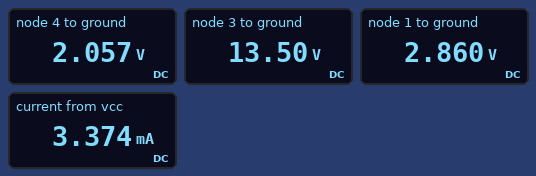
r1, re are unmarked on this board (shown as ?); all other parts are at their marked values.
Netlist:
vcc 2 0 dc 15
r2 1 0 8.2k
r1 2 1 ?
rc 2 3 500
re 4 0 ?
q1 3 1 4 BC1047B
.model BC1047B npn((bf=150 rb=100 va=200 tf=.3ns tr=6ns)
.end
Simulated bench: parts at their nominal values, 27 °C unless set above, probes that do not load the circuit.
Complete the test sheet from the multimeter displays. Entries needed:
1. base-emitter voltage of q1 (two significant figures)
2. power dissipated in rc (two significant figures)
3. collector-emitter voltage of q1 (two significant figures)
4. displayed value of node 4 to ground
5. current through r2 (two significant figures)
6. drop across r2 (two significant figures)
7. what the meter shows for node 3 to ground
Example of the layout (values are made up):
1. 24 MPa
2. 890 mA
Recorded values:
1. 800 mV
2. 4.5 mW
3. 11 V
4. 2.057 V
5. 350 µA
6. 2.9 V
7. 13.50 V
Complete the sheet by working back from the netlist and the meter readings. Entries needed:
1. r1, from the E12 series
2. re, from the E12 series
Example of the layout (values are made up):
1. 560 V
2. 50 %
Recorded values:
1. 33 kΩ
2. 680 Ω
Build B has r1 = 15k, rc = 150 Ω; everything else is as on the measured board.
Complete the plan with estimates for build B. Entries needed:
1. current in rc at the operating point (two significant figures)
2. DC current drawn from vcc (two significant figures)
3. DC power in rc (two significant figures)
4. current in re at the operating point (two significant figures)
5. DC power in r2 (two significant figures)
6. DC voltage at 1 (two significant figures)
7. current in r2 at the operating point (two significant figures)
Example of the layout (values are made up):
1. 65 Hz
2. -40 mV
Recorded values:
1. 6.2 mA
2. 6.9 mA
3. 5.8 mW
4. 6.3 mA
5. 3.2 mW
6. 5.1 V
7. 620 µA
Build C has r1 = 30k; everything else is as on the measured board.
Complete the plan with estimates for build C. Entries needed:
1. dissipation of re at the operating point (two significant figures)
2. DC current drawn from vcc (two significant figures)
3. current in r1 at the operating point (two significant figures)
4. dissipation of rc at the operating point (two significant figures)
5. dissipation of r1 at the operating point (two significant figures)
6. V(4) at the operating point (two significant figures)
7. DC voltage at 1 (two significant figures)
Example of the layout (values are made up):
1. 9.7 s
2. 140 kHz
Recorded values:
1. 7.6 mW
2. 3.7 mA
3. 400 µA
4. 5.5 mW
5. 4.7 mW
6. 2.3 V
7. 3.1 V
